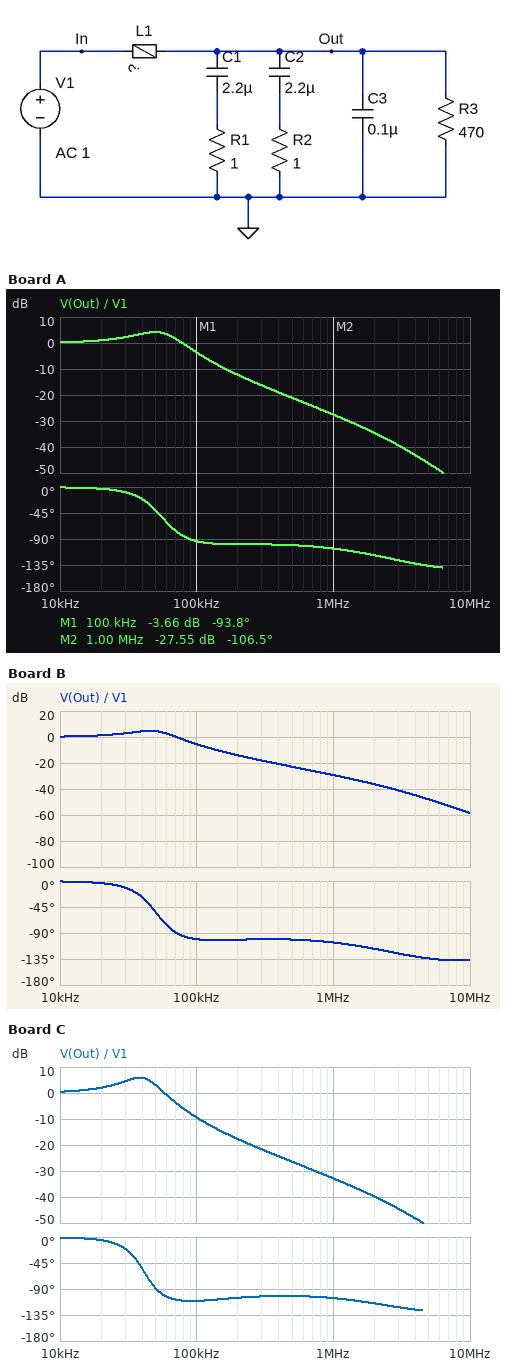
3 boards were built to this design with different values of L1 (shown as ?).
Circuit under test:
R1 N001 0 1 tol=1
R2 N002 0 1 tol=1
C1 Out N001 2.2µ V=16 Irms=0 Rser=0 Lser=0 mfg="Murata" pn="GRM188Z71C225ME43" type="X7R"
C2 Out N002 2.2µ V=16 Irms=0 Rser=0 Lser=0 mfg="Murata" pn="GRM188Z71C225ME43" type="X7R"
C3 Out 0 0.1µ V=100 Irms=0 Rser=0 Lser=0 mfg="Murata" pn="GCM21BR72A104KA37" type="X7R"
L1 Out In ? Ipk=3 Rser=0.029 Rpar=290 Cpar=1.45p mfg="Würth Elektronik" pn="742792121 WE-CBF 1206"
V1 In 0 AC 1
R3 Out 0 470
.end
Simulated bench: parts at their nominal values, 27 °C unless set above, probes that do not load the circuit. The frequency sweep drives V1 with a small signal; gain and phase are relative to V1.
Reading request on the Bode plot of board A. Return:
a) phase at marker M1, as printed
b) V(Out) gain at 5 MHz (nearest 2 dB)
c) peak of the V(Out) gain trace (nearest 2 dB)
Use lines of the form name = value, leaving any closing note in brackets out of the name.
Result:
phase at marker M1, as printed = -93.8 deg
V(Out) gain at 5 MHz = -46 dB
peak of the V(Out) gain trace = 4 dB
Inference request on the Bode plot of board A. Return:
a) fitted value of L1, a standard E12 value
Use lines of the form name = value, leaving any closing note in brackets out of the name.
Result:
fitted value of L1, a standard E12 value = 1.8 µH
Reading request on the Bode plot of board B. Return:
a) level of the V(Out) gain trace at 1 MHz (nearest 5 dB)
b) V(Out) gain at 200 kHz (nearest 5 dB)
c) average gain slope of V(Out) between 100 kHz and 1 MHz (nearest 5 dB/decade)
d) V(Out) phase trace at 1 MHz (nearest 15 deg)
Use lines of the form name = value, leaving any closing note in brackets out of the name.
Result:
level of the V(Out) gain trace at 1 MHz = -30 dB
V(Out) gain at 200 kHz = -15 dB
average gain slope of V(Out) between 100 kHz and 1 MHz = -25 dB/decade
V(Out) phase trace at 1 MHz = -105 deg
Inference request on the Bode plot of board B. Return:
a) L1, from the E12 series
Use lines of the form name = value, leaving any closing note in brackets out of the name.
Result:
L1, from the E12 series = 2.2 µH
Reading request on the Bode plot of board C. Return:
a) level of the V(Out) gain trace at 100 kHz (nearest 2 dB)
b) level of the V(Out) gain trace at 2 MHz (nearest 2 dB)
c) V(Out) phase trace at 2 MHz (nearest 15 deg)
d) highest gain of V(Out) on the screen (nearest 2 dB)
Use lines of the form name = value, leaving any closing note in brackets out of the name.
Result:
level of the V(Out) gain trace at 100 kHz = -10 dB
level of the V(Out) gain trace at 2 MHz = -40 dB
V(Out) phase trace at 2 MHz = -120 deg
highest gain of V(Out) on the screen = 6 dB
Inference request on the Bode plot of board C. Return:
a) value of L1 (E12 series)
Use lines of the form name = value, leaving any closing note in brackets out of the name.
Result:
value of L1 = 3.3 µH
